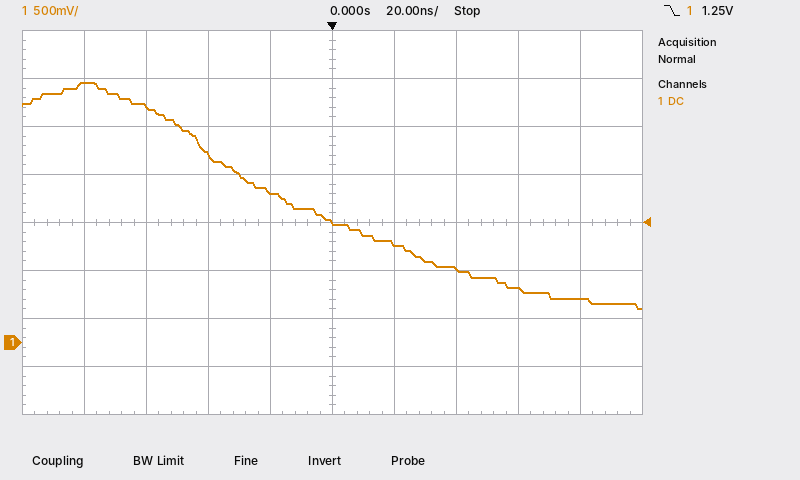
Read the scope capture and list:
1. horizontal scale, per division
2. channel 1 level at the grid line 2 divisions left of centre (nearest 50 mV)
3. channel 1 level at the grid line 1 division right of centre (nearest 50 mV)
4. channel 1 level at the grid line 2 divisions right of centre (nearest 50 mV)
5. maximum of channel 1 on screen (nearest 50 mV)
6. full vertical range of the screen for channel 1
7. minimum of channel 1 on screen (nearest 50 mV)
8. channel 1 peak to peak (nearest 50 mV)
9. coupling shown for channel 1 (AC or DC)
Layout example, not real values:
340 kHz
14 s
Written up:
20 ns
1.95 V
1.05 V
750 mV
2.70 V
4 V
350 mV
2.35 V
DC
